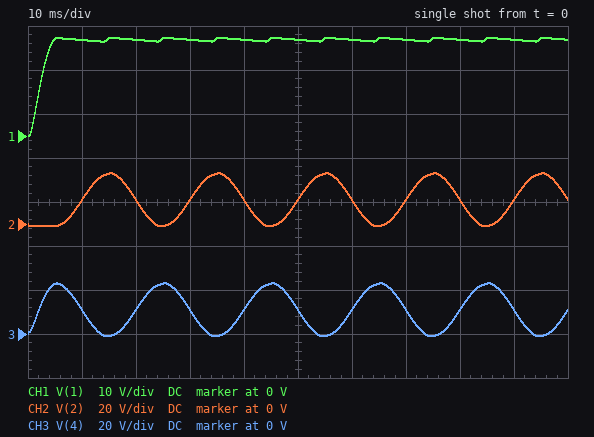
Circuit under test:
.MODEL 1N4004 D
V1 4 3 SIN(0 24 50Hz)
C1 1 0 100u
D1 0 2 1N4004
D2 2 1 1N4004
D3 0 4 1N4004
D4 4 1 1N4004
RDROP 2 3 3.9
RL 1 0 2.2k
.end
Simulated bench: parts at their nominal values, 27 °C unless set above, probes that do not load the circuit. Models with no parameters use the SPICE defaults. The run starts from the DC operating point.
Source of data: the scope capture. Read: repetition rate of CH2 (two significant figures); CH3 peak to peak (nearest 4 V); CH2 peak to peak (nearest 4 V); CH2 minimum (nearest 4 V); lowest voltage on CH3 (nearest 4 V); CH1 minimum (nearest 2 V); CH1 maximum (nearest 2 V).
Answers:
50 Hz
24 V
24 V
0 V
0 V
0 V
22 V
